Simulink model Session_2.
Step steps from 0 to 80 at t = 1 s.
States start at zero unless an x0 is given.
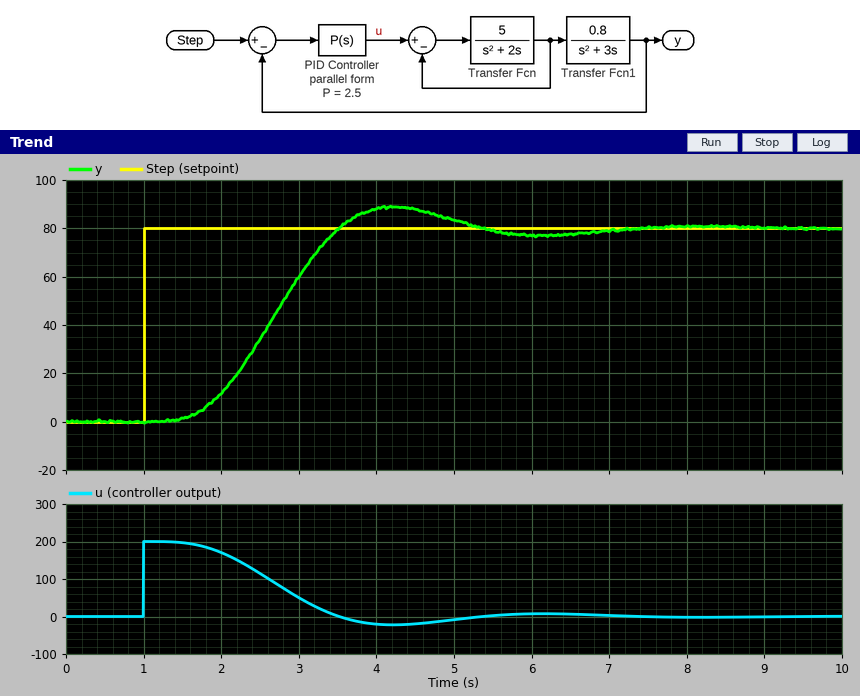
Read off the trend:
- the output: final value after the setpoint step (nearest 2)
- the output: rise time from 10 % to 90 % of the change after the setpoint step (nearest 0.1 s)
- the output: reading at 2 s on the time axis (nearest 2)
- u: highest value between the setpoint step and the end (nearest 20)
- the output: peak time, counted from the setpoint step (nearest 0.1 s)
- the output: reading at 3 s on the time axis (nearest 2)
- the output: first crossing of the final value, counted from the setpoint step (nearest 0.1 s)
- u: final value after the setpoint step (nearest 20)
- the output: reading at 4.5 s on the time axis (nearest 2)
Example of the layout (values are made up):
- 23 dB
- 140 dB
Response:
- 80
- 1.4 s
- 12
- 200
- 3.2 s
- 60
- 2.5 s
- 0
- 88
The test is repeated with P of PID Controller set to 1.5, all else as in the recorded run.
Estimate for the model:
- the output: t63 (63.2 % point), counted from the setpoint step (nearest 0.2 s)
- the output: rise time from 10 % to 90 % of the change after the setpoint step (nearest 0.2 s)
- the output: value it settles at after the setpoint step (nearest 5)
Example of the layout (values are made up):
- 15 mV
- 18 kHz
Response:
- 2.4 s
- 3.6 s
- 80
